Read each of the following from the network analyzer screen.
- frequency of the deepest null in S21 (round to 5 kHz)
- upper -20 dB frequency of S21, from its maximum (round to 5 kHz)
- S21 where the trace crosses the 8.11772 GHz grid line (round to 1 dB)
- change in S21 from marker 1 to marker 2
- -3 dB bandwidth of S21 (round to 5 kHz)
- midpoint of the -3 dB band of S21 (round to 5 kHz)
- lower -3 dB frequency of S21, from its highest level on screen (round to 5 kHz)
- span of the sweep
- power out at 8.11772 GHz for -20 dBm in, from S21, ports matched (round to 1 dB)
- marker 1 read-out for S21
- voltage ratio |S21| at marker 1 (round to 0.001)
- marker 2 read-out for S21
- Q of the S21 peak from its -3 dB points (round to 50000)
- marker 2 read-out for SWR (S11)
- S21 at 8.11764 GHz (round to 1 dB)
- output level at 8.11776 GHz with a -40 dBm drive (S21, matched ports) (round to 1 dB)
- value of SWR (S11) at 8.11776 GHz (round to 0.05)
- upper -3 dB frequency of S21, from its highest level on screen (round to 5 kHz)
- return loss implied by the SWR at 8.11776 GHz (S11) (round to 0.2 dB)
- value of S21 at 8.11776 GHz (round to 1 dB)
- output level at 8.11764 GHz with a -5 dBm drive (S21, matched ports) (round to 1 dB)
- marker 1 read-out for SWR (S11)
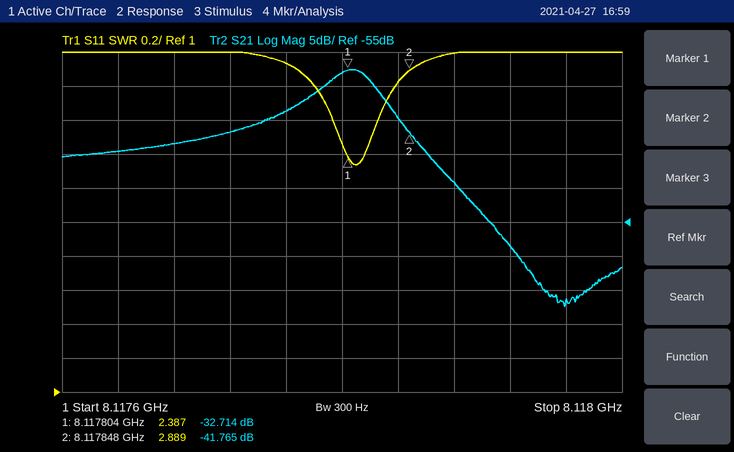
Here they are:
8.117960 GHz
8.117895 GHz
-42 dB
-9.051 dB
40 kHz
8.117805 GHz
8.117785 GHz
400 kHz
-62 dBm
-32.714 dB
0.023
-41.765 dB
200000
2.889
-45 dB
-79 dBm
2.95
8.117825 GHz
6.2 dB
-39 dB
-50 dBm
2.387
